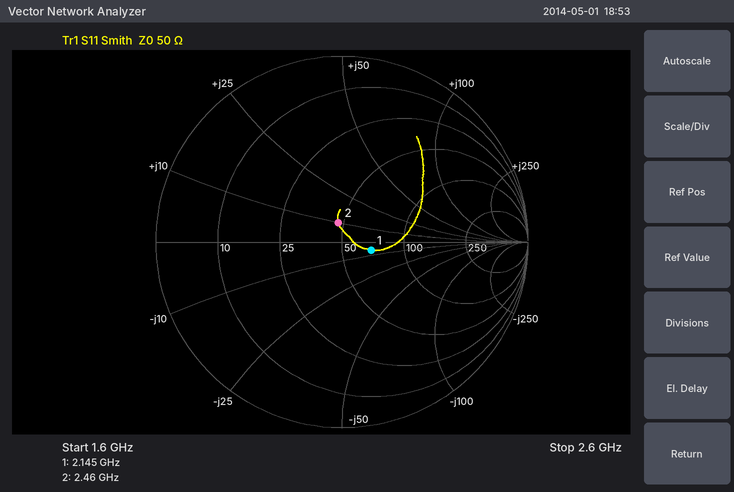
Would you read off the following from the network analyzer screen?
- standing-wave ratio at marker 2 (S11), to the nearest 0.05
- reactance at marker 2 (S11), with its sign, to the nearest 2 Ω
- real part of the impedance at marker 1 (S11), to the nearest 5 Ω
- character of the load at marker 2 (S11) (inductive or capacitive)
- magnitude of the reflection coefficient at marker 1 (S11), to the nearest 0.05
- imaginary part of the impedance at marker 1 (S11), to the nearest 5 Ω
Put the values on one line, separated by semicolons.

1.25; +10 Ω; 70 Ω; inductive; 0.15; -5 Ω
